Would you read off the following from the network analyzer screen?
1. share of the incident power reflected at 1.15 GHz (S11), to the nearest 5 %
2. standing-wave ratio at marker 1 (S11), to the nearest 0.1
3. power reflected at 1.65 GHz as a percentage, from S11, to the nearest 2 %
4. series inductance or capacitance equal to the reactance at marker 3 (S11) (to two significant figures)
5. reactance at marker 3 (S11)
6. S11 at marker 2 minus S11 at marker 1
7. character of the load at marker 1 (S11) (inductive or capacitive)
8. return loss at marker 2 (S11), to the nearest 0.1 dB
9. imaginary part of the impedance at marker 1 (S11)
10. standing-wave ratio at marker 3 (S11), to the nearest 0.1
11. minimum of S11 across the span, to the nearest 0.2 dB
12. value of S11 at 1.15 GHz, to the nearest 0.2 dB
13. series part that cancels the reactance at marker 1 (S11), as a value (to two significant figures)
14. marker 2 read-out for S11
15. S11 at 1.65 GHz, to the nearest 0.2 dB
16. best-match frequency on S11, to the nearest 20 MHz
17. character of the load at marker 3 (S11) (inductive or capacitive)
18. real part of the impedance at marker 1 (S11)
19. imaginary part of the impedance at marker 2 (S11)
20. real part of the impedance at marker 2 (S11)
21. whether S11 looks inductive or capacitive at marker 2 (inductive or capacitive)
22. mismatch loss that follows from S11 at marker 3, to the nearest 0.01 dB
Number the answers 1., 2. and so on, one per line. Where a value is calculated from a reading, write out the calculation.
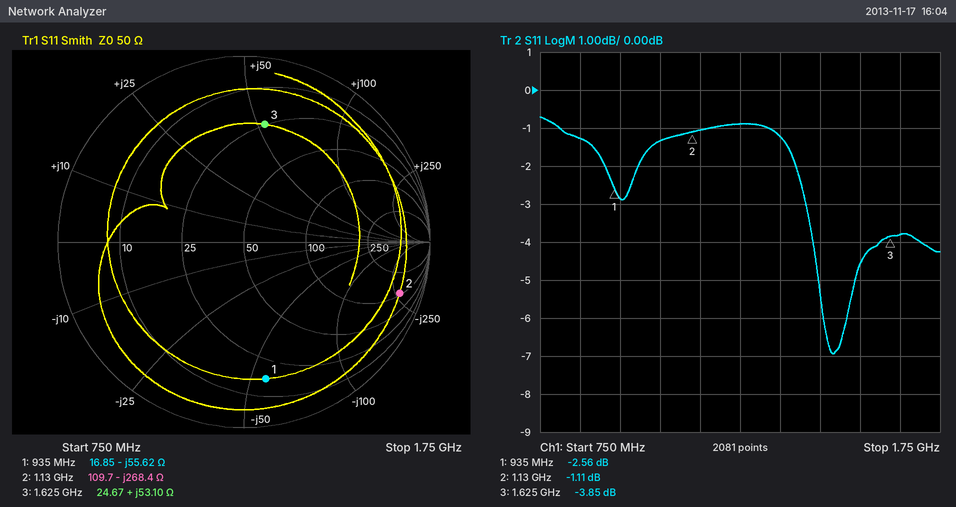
1. 10^(-1/10) ≈ 79.4 %, so 80 % to the nearest 5 %
2. 6.8
3. 10^(-3.8/10) ≈ 42 %
4. L = 53.1 Ω/(2π × 1.625 GHz) ≈ 5.2 nH
5. +53.10 Ω
6. -1.11 − (-2.56) = 1.45 dB
7. capacitive
8. 1.1 dB
9. -55.62 Ω
10. 4.6
11. -7.0 dB
12. -1.0 dB
13. L = 55.62 Ω/(2π × 935 MHz) ≈ 9.5 nH
14. -1.11 dB
15. -3.8 dB
16. 1.48 GHz
17. inductive
18. 16.85 Ω
19. -268.4 Ω
20. 109.7 Ω
21. capacitive
22. −10 log10(1 − 10^(-3.85/10)) ≈ 2.31 dB
